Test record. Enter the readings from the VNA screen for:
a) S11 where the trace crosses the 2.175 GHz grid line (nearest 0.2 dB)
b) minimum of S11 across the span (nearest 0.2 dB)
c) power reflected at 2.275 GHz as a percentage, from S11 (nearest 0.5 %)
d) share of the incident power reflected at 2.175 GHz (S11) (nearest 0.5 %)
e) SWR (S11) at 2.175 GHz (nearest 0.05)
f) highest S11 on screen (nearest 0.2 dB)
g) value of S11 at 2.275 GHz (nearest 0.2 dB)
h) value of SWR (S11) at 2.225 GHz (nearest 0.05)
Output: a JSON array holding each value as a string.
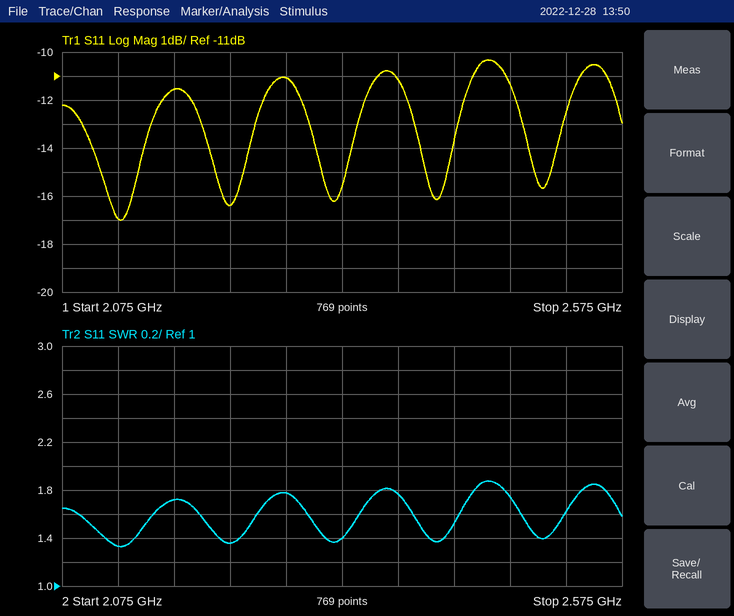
["-11.6 dB", "-17.0 dB", "8.0 %", "7.0 %", "1.70", "-10.4 dB", "-11.0 dB", "1.35"]
